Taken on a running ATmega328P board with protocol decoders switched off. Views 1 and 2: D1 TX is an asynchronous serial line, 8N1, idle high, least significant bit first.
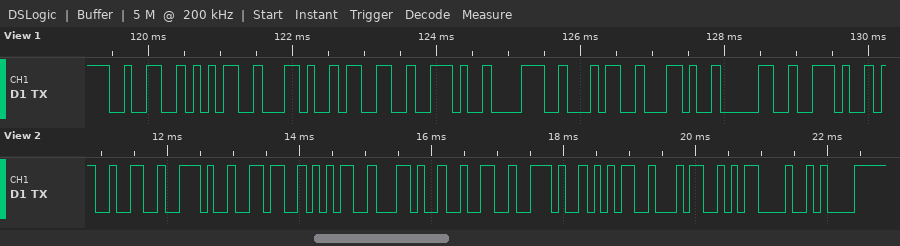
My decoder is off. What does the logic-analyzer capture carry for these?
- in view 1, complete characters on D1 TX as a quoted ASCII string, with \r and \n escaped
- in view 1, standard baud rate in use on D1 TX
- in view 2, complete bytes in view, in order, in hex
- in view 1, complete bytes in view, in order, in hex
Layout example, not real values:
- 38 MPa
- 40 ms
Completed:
- "25,3.84,0."
- 9600 baud
- 32 2E 36 35 2C 32 2E 35 34 0D 0A
- 32 35 2C 33 2E 38 34 2C 30 2E
